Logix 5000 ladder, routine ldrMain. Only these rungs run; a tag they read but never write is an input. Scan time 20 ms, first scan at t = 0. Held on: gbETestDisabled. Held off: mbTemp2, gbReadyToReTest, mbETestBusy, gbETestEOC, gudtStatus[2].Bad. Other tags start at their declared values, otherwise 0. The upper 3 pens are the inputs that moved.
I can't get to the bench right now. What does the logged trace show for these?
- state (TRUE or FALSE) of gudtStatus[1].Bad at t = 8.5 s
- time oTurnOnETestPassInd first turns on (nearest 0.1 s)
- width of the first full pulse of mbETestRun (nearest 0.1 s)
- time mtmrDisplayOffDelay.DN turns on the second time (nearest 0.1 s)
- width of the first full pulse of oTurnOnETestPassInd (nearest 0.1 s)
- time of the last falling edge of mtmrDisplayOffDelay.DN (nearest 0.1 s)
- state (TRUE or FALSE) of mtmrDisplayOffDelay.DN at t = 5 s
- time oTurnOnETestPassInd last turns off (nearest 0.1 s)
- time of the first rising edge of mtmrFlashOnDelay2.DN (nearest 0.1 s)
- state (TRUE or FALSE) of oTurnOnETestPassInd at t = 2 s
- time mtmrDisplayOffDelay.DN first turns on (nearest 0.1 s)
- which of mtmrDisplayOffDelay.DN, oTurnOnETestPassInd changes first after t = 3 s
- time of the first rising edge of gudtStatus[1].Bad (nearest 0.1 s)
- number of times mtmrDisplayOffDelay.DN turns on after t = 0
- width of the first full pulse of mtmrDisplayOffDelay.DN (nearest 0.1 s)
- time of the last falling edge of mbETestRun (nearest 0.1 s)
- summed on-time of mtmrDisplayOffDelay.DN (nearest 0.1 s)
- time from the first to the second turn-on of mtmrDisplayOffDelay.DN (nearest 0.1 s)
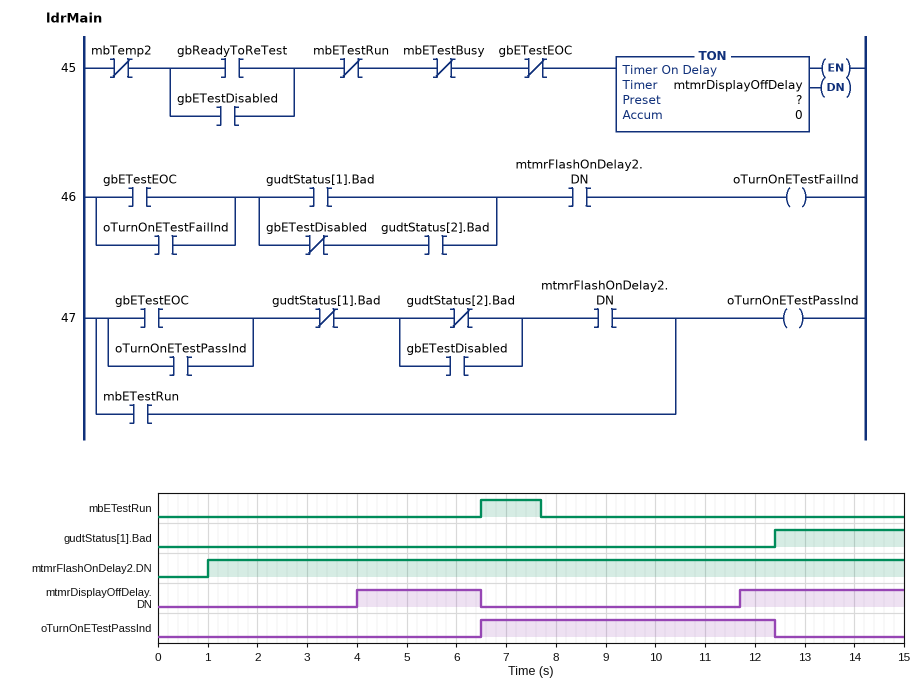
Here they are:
FALSE
6.5 s
1.2 s
11.7 s
5.9 s
6.5 s
TRUE
12.4 s
1.0 s
FALSE
4.0 s
mtmrDisplayOffDelay.DN
12.4 s
2
2.5 s
7.7 s
5.8 s
7.7 s
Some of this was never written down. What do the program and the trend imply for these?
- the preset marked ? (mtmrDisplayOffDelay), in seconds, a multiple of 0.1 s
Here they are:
4.0 s
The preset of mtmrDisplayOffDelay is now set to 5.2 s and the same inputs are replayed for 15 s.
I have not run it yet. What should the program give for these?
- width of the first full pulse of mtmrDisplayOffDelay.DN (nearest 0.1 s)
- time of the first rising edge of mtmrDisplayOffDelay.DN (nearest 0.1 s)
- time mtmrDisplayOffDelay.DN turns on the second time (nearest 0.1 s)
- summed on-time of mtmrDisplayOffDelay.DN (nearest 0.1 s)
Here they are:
1.3 s
5.2 s
12.9 s
3.4 s
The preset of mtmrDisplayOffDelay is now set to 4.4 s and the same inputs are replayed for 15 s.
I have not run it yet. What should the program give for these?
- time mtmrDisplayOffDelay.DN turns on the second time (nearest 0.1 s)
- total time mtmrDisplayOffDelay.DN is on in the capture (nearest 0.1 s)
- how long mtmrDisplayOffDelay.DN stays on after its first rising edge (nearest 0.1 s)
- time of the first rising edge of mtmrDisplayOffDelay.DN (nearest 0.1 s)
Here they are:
12.1 s
5.0 s
2.1 s
4.4 s
